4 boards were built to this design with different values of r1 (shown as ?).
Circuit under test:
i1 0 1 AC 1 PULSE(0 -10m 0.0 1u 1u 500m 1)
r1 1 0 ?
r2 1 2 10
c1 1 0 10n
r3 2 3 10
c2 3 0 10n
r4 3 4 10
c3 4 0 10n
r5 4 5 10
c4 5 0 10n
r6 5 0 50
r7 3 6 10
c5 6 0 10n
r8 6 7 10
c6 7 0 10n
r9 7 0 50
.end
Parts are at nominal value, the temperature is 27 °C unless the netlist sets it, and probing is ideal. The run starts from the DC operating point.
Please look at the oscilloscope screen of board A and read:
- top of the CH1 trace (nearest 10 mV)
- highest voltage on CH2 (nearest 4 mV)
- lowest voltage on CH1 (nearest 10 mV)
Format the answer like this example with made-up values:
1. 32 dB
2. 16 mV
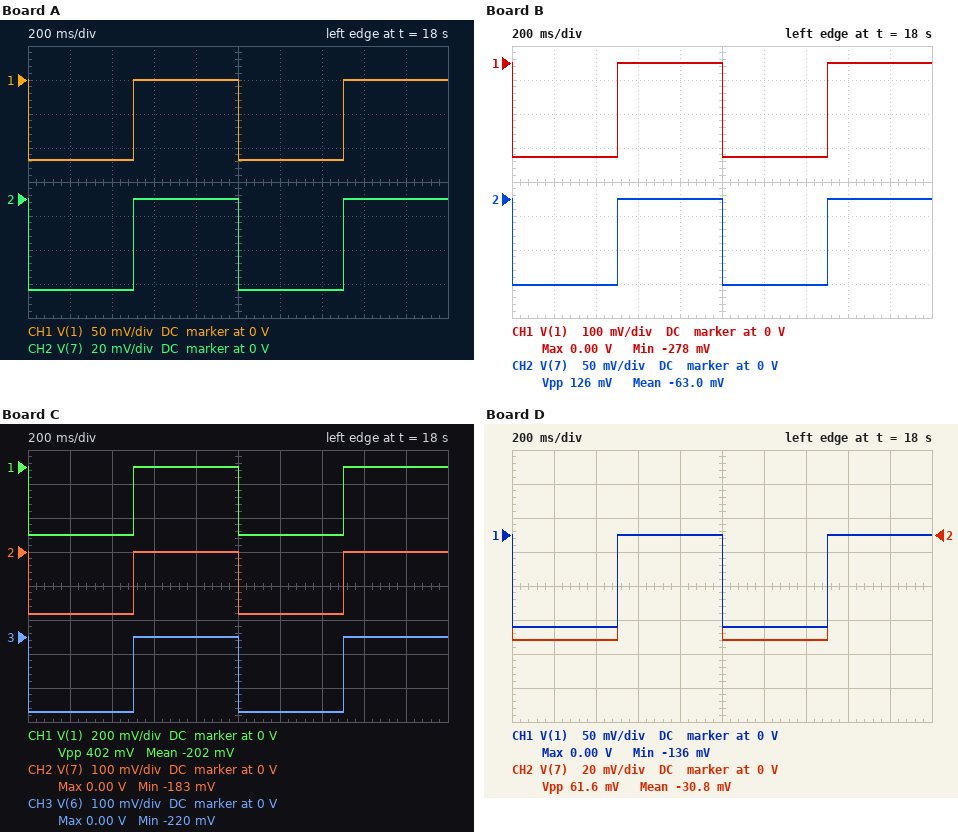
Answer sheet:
1. 0 V
2. 0 V
3. -120 mV
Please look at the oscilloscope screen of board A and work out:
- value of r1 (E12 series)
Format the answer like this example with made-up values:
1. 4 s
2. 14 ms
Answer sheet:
1. 15 Ω
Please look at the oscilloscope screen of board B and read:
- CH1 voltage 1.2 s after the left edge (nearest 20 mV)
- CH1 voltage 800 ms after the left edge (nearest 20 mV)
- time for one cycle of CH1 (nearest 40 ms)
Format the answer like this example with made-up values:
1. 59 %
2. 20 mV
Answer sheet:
1. -280 mV
2. 0 V
3. 1.00 s
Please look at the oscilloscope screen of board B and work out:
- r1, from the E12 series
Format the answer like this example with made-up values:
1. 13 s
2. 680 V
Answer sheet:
1. 56 Ω
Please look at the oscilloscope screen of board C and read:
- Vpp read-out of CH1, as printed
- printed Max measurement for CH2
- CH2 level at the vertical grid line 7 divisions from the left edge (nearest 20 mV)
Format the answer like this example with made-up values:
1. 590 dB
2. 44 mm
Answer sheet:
1. 402 mV
2. 0.00 V
3. -180 mV
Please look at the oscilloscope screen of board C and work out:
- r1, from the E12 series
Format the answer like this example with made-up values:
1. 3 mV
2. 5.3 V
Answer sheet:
1. 150 Ω
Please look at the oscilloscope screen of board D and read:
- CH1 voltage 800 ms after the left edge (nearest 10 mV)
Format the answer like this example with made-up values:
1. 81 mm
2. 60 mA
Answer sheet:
1. 0 V
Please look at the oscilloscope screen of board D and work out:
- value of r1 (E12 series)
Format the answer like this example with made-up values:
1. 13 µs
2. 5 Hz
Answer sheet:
1. 18 Ω
